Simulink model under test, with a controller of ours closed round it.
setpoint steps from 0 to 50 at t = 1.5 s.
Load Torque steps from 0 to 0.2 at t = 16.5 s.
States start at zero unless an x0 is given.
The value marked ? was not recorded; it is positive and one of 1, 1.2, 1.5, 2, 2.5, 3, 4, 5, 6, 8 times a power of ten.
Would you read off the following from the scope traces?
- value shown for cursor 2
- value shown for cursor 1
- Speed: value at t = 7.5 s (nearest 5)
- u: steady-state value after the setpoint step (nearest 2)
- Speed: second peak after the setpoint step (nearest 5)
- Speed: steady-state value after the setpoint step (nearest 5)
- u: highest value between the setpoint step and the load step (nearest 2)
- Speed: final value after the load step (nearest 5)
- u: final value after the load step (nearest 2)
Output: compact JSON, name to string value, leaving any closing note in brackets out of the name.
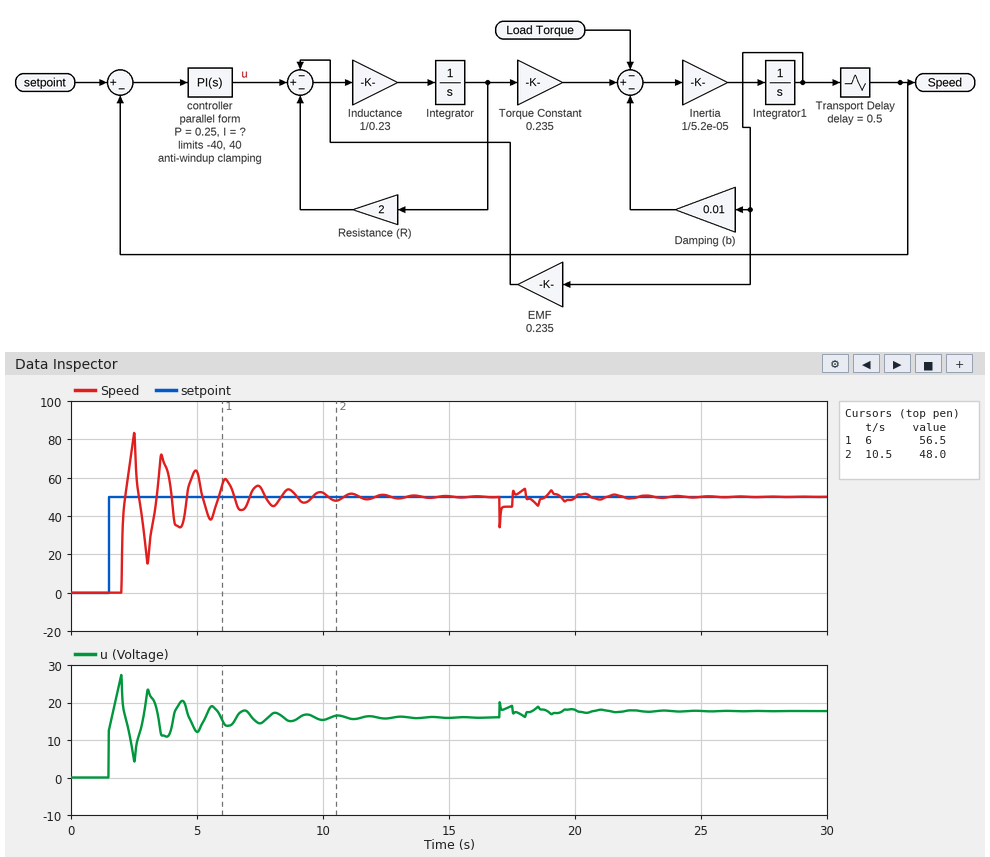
{"value shown for cursor 2": "48.0", "value shown for cursor 1": "56.5", "Speed: value at t = 7.5 s": "55", "u: steady-state value after the setpoint step": "16", "Speed: second peak after the setpoint step": "70", "Speed: steady-state value after the setpoint step": "50", "u: highest value between the setpoint step and the load step": "28", "Speed: final value after the load step": "50", "u: final value after the load step": "18"}
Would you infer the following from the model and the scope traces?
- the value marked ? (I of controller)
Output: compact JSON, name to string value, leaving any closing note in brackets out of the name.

{"the value marked ?": "0.6"}
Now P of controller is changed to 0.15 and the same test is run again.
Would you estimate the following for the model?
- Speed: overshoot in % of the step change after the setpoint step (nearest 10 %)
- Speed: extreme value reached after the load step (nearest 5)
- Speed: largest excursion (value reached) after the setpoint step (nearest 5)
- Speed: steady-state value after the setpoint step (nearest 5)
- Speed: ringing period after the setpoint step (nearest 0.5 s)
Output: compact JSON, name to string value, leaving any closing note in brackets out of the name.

{"Speed: overshoot in % of the step change after the setpoint step": "40 %", "Speed: extreme value reached after the load step": "35", "Speed: largest excursion (value reached) after the setpoint step": "70", "Speed: steady-state value after the setpoint step": "50", "Speed: ringing period after the setpoint step": "1.5 s"}
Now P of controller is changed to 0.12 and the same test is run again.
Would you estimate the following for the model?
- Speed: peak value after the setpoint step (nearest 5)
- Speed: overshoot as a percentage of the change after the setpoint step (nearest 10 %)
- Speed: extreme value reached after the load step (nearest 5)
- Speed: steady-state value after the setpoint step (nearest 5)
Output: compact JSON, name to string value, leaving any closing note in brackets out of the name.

{"Speed: peak value after the setpoint step": "65", "Speed: overshoot as a percentage of the change after the setpoint step": "30 %", "Speed: extreme value reached after the load step": "35", "Speed: steady-state value after the setpoint step": "50"}
